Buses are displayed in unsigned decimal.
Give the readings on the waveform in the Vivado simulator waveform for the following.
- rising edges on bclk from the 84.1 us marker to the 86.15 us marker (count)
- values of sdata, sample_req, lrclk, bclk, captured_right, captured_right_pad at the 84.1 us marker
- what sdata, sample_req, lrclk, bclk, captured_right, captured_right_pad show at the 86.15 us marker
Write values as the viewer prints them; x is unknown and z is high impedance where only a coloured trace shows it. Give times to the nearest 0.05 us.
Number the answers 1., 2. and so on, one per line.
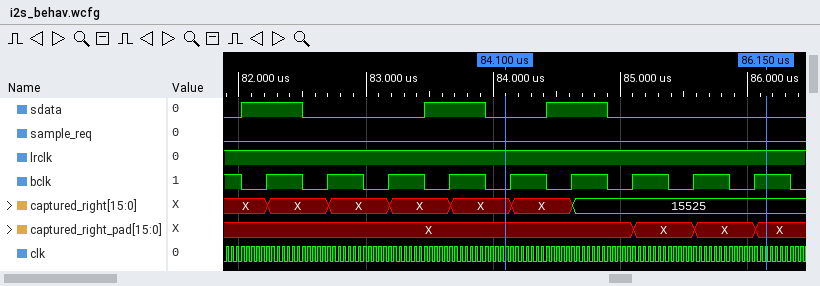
1. 5
2. sdata=0, sample_req=0, lrclk=1, bclk=0, captured_right=X, captured_right_pad=X
3. sdata=0, sample_req=0, lrclk=1, bclk=1, captured_right=15525, captured_right_pad=X
